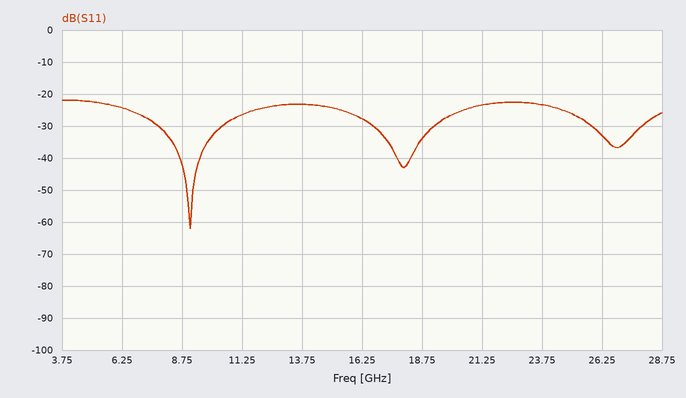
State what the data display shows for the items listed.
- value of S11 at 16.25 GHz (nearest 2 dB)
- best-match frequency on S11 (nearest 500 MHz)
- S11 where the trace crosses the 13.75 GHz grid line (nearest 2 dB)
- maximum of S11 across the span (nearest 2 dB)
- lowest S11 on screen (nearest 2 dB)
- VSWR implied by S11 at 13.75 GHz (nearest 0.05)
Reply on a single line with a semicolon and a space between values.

-28 dB; 9.0 GHz; -24 dB; -22 dB; -62 dB; 1.15
